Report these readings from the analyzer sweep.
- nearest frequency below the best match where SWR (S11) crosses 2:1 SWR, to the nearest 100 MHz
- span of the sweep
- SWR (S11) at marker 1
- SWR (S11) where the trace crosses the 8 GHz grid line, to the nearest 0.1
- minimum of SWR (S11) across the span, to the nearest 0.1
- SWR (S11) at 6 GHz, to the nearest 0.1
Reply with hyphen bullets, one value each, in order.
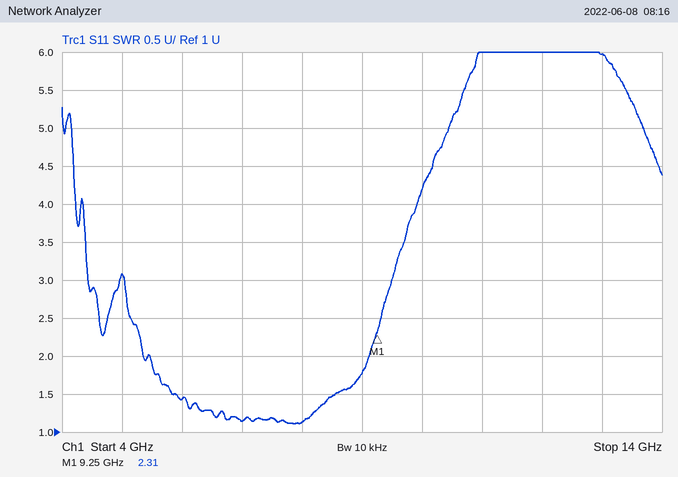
- 5.5 GHz
- 10 GHz
- 2.31
- 1.1
- 1.1
- 1.4
